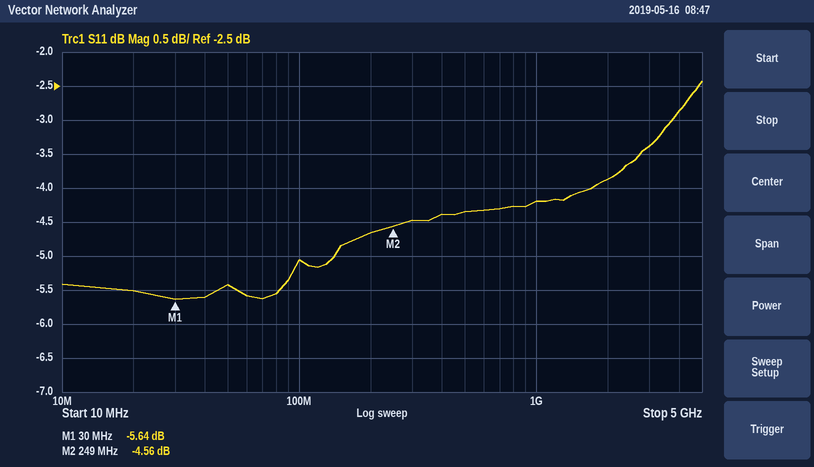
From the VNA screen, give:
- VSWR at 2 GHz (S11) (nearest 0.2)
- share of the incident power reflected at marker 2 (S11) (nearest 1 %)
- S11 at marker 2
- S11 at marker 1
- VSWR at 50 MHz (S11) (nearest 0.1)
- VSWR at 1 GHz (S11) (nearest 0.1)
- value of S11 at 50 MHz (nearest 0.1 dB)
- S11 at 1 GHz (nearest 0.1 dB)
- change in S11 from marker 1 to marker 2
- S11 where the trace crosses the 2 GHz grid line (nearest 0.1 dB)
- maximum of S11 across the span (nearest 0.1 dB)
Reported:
4.6
35 %
-4.56 dB
-5.64 dB
3.3
4.2
-5.4 dB
-4.2 dB
1.08 dB
-3.9 dB
-2.4 dB
